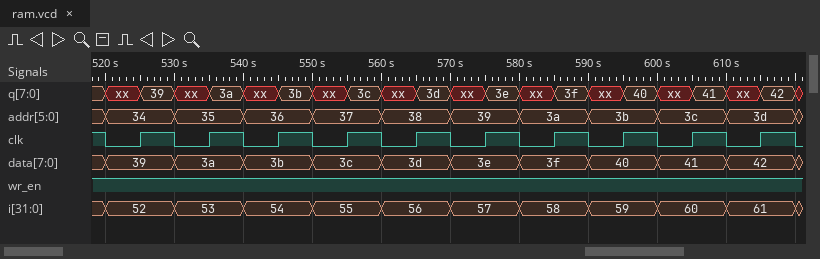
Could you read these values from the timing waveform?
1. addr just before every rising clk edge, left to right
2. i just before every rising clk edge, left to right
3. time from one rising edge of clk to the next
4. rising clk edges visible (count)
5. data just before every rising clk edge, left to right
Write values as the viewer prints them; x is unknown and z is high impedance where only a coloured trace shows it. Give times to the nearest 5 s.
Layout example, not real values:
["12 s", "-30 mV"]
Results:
["34, 35, 36, 37, 38, 39, 3a, 3b, 3c, 3d", "52, 53, 54, 55, 56, 57, 58, 59, 60, 61", "10 s", "10", "39, 3a, 3b, 3c, 3d, 3e, 3f, 40, 41, 42"]
